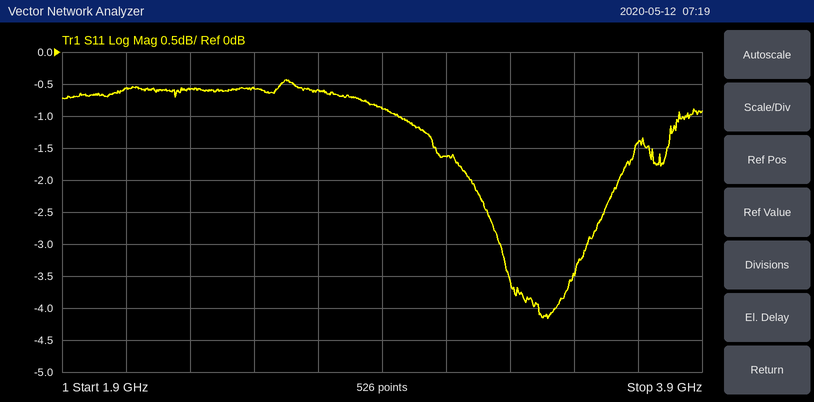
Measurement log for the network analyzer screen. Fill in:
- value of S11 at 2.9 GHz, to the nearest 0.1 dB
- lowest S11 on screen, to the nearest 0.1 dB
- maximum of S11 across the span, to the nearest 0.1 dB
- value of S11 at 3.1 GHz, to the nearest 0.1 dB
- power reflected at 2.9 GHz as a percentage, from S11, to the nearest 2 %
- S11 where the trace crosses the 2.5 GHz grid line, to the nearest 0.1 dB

-0.9 dB
-4.2 dB
-0.4 dB
-1.6 dB
82 %
-0.6 dB
